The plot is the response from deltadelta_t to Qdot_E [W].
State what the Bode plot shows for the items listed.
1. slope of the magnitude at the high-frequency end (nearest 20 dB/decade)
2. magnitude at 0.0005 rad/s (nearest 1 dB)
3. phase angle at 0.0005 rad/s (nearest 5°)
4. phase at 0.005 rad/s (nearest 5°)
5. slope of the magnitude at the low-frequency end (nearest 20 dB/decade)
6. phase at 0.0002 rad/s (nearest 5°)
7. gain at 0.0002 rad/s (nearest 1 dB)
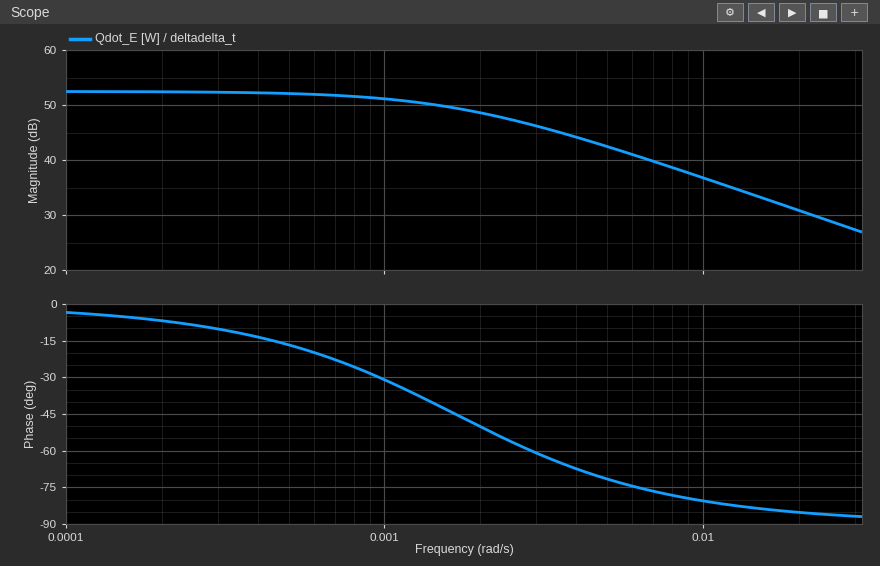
-20 dB/decade
52 dB
-15°
-70°
0 dB/decade
-5°
52 dB
